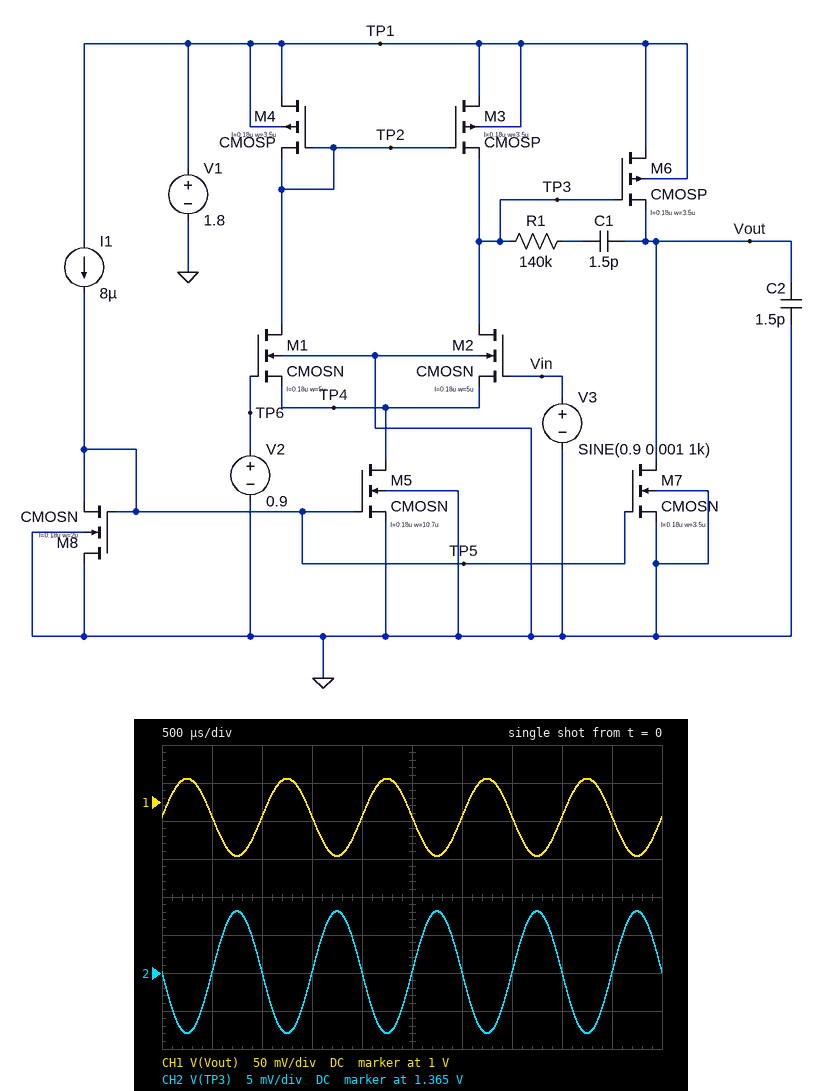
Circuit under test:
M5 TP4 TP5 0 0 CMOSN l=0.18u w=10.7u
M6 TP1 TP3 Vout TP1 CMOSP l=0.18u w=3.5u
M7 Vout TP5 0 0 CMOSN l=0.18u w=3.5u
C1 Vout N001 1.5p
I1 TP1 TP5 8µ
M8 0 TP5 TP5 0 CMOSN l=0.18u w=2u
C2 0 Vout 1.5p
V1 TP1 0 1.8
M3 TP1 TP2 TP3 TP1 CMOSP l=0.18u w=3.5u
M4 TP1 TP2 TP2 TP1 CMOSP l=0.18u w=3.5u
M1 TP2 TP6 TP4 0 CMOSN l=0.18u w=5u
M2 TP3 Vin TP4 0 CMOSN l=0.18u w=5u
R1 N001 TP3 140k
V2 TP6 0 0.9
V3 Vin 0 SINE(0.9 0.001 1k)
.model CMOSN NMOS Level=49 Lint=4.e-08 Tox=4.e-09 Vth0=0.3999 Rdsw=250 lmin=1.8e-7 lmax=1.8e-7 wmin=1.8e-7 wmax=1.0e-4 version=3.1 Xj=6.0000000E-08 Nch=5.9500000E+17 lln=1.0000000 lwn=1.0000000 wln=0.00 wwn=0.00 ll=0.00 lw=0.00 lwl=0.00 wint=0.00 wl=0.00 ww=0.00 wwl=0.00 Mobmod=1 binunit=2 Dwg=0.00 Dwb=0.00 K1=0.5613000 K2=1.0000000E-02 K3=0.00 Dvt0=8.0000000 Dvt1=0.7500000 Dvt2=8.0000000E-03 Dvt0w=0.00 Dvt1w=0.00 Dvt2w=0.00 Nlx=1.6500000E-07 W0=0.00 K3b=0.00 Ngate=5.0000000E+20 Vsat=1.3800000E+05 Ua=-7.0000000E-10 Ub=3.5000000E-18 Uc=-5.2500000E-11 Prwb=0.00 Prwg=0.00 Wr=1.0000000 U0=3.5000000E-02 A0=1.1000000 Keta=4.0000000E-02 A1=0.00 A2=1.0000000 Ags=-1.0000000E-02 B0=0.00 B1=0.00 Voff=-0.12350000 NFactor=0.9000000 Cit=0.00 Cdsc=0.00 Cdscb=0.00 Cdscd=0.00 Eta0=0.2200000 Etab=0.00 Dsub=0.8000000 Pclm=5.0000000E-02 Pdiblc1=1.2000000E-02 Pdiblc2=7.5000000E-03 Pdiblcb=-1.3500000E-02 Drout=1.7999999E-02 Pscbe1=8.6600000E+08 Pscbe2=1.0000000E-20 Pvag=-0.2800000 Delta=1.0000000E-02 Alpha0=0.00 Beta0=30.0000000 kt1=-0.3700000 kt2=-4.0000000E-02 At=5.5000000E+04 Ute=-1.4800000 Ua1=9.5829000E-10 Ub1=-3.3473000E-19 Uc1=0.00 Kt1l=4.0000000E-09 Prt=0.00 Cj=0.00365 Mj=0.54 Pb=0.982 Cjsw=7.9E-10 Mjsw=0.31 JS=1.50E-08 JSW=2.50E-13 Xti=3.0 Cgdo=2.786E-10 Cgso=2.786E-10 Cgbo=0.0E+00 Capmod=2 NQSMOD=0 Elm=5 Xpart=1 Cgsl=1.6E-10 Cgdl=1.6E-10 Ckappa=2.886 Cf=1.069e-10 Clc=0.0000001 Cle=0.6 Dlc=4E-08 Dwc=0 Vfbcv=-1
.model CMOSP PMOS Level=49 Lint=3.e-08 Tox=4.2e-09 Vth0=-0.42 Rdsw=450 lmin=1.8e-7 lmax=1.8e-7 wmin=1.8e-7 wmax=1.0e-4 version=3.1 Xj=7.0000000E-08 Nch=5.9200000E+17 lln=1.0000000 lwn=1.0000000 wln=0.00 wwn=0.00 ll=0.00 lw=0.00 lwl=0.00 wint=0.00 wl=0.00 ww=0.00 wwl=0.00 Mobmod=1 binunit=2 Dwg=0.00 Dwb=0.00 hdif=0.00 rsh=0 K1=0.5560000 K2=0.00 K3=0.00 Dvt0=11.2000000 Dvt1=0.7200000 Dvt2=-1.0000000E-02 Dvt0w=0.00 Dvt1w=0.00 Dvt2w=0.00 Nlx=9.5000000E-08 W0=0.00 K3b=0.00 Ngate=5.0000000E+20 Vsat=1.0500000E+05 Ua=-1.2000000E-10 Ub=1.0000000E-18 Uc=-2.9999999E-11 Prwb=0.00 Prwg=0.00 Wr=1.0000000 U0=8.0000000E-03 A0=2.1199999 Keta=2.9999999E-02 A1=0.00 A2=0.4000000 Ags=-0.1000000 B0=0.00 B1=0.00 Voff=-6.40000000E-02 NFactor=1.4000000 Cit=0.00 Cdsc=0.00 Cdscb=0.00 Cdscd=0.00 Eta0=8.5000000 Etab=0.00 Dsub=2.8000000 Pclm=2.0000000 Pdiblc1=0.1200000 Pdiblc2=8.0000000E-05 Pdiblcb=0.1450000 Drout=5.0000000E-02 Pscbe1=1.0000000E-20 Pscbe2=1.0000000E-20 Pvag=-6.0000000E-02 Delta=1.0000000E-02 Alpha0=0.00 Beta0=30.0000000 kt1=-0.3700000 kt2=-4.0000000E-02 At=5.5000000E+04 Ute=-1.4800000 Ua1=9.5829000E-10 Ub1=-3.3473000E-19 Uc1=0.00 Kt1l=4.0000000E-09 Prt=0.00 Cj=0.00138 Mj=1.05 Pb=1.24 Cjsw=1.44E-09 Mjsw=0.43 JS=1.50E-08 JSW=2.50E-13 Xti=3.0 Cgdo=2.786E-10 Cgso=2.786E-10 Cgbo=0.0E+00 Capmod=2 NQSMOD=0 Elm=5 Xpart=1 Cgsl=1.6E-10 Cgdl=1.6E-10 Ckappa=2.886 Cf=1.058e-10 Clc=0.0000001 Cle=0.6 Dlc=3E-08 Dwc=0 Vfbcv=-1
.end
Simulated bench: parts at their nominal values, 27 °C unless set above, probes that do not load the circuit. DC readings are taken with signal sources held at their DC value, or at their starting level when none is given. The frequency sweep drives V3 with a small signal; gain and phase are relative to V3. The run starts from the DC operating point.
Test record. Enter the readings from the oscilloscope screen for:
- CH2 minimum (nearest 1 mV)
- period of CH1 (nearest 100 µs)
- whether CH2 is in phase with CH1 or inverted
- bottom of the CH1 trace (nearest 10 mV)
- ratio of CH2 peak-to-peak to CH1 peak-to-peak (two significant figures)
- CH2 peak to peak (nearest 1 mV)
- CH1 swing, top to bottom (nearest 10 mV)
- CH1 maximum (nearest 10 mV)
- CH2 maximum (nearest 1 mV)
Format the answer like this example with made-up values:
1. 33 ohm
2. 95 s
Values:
1. 1.357 V
2. 1.0 ms
3. inverted
4. 930 mV
5. 0.16
6. 16 mV
7. 100 mV
8. 1.03 V
9. 1.373 V
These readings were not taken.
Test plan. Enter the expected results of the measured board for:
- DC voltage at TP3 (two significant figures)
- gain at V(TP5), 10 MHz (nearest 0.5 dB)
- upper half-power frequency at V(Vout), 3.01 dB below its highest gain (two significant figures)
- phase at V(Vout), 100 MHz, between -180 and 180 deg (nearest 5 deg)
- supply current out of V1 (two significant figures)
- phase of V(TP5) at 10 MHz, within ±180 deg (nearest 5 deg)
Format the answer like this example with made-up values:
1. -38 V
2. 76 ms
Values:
1. 1.4 V
2. -39.0 dB
3. 410 kHz
4. -100 deg
5. 83 µA
6. 45 deg
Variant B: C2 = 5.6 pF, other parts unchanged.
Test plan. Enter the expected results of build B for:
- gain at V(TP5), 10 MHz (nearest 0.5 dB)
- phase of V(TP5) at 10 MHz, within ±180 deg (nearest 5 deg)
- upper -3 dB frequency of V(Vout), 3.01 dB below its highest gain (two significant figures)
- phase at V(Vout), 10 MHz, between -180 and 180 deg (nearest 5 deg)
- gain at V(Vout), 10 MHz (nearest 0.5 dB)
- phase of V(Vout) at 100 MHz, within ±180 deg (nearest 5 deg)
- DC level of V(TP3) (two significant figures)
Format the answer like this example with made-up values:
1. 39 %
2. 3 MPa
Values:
1. -47.0 dB
2. 20 deg
3. 360 kHz
4. -75 deg
5. 16.0 dB
6. -105 deg
7. 1.4 V
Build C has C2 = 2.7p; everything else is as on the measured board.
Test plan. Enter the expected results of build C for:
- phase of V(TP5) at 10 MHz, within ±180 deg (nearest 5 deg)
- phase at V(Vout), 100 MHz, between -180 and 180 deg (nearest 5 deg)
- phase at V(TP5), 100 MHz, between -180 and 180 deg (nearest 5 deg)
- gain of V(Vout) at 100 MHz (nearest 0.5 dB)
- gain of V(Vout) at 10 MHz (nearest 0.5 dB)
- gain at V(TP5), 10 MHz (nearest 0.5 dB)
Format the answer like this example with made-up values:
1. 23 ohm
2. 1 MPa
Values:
1. 30 deg
2. -105 deg
3. 10 deg
4. 2.5 dB
5. 21.5 dB
6. -42.0 dB
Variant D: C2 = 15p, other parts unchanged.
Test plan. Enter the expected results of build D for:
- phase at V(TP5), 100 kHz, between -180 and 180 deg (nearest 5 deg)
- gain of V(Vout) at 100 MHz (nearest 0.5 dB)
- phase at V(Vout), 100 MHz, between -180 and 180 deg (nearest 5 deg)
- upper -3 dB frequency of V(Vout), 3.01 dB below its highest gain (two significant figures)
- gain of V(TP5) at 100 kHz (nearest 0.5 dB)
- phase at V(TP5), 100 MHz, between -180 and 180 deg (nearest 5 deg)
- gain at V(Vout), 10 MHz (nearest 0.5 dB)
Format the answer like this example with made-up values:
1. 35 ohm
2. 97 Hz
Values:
1. 70 deg
2. -12.5 dB
3. -105 deg
4. 270 kHz
5. -70.0 dB
6. 80 deg
7. 8.0 dB
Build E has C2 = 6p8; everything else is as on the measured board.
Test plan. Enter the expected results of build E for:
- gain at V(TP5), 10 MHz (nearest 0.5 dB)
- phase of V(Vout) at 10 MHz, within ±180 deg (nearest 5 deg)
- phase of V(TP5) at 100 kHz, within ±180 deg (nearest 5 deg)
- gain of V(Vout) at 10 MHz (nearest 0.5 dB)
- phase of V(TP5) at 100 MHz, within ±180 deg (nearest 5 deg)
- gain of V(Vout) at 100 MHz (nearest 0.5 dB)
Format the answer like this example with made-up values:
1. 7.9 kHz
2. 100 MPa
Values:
1. -48.5 dB
2. -80 deg
3. 75 deg
4. 14.5 dB
5. 50 deg
6. -5.5 dB
